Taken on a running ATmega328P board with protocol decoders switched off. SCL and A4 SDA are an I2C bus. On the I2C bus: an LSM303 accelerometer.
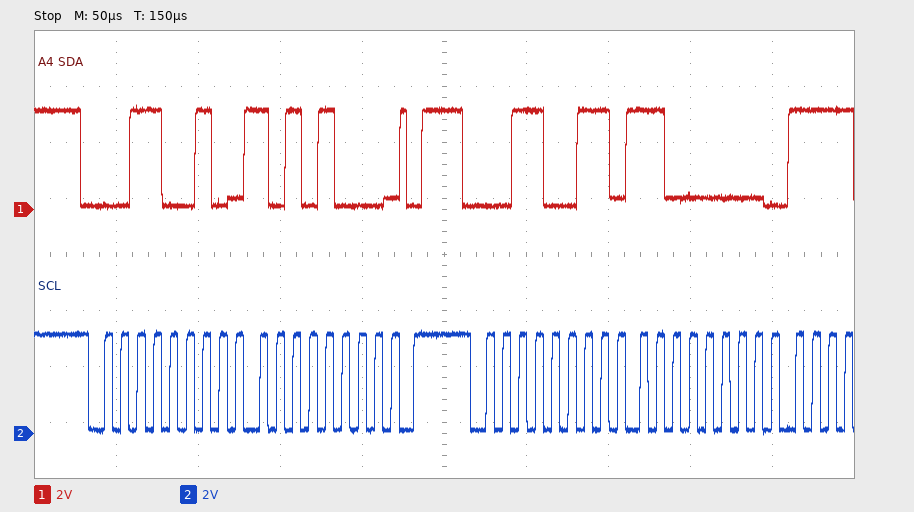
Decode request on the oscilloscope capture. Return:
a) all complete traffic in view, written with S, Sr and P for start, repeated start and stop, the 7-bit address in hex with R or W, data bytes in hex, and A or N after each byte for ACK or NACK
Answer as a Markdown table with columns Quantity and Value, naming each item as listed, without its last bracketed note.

| Quantity | Value |
|---|---|
| all complete traffic in view, written with S, Sr and P for start, repeated start and stop, the 7-bit address in hex with R or W, data bytes in hex, and A or N after each byte for ACK or NACK | S 19W A A8 A P S 19R A C0 A |
